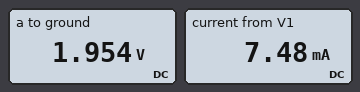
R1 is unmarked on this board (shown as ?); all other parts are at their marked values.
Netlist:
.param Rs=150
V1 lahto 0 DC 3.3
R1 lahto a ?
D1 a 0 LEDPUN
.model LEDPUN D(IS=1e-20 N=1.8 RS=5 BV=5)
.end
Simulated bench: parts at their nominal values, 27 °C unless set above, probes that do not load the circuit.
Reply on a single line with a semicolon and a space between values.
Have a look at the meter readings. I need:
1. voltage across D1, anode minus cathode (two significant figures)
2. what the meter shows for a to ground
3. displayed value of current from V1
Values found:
2.0 V; 1.954 V; 7.48 mA
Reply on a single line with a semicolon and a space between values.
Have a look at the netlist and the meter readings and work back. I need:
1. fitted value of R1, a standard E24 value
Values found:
180 Ω
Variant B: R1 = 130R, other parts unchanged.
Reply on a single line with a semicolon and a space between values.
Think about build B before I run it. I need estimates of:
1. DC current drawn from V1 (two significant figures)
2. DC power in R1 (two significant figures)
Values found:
10 mA; 13 mW
